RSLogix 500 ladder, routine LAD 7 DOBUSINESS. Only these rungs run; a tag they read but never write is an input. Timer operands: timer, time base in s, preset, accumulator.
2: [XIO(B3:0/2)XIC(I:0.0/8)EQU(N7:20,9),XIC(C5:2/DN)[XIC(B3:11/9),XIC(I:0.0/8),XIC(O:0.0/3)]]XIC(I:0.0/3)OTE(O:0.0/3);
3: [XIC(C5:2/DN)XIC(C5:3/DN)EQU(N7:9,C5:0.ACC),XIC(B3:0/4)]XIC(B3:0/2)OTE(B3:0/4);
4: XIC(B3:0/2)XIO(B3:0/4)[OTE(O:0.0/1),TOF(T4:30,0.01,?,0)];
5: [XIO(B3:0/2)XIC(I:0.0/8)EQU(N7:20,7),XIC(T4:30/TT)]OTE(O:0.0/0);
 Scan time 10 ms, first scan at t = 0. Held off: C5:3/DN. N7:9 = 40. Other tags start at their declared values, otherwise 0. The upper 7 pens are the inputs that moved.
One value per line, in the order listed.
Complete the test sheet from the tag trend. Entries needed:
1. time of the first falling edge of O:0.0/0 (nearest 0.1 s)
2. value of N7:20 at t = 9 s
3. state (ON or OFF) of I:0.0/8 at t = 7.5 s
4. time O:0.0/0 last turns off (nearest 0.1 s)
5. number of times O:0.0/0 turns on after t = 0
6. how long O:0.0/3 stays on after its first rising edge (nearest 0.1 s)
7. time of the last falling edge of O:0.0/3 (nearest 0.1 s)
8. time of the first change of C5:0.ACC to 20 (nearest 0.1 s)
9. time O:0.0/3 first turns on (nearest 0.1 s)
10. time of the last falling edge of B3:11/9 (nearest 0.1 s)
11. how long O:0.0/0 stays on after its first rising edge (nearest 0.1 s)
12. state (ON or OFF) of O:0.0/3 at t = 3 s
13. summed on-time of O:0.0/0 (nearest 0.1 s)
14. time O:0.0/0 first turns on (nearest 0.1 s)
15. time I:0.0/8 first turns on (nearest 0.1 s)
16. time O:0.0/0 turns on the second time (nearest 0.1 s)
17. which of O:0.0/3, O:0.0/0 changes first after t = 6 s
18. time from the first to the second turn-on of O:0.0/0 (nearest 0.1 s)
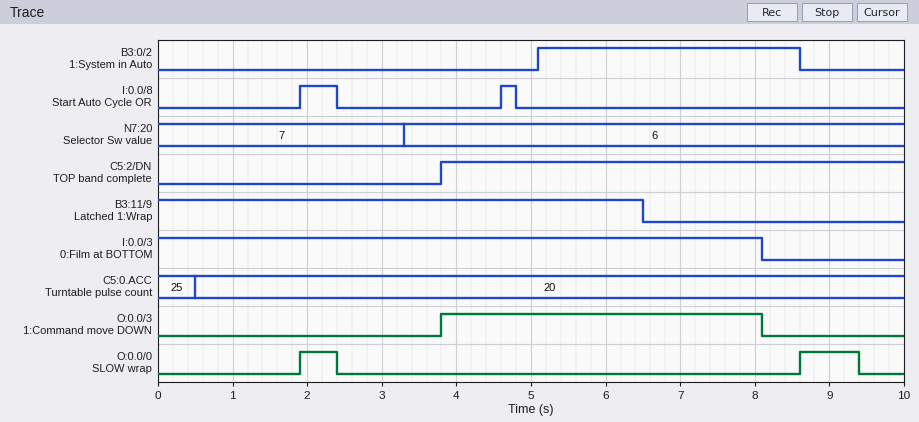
2.4 s
6
OFF
9.4 s
2
4.3 s
8.1 s
0.5 s
3.8 s
6.5 s
0.5 s
OFF
1.3 s
1.9 s
1.9 s
8.6 s
O:0.0/3
6.7 s
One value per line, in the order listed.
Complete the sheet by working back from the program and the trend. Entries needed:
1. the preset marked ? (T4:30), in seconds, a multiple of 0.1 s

0.8 s
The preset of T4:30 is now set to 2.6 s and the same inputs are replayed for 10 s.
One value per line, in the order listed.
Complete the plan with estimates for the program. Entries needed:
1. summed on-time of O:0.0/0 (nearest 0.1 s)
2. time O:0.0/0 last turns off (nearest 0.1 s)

1.9 s
2.4 s
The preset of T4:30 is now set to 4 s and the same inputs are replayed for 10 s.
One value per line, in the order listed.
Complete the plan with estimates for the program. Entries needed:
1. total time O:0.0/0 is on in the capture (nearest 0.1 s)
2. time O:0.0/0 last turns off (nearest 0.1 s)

1.9 s
2.4 s
